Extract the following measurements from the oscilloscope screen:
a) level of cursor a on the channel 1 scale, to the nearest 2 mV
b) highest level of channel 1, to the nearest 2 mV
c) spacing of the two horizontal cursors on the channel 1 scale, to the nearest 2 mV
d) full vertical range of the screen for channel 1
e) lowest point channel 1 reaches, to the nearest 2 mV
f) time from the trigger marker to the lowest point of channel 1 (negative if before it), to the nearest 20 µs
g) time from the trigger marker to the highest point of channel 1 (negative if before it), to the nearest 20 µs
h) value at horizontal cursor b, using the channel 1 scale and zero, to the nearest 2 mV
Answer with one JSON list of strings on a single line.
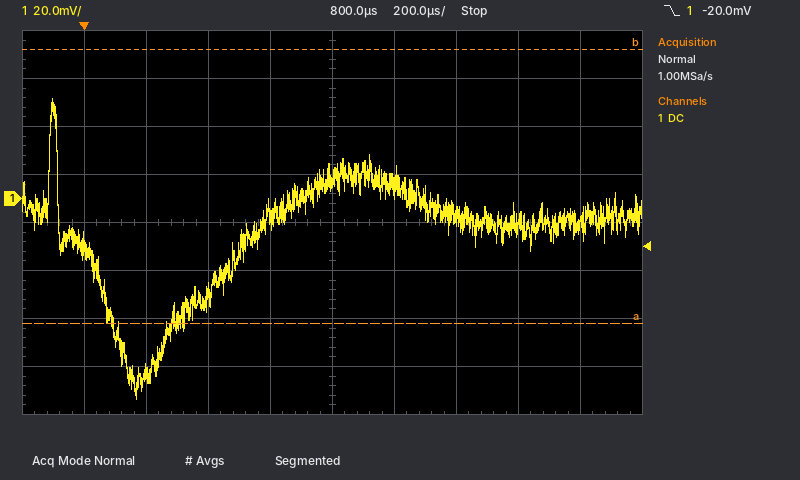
["-52 mV", "42 mV", "114 mV", "160 mV", "-84 mV", "+160 µs", "-100 µs", "62 mV"]
